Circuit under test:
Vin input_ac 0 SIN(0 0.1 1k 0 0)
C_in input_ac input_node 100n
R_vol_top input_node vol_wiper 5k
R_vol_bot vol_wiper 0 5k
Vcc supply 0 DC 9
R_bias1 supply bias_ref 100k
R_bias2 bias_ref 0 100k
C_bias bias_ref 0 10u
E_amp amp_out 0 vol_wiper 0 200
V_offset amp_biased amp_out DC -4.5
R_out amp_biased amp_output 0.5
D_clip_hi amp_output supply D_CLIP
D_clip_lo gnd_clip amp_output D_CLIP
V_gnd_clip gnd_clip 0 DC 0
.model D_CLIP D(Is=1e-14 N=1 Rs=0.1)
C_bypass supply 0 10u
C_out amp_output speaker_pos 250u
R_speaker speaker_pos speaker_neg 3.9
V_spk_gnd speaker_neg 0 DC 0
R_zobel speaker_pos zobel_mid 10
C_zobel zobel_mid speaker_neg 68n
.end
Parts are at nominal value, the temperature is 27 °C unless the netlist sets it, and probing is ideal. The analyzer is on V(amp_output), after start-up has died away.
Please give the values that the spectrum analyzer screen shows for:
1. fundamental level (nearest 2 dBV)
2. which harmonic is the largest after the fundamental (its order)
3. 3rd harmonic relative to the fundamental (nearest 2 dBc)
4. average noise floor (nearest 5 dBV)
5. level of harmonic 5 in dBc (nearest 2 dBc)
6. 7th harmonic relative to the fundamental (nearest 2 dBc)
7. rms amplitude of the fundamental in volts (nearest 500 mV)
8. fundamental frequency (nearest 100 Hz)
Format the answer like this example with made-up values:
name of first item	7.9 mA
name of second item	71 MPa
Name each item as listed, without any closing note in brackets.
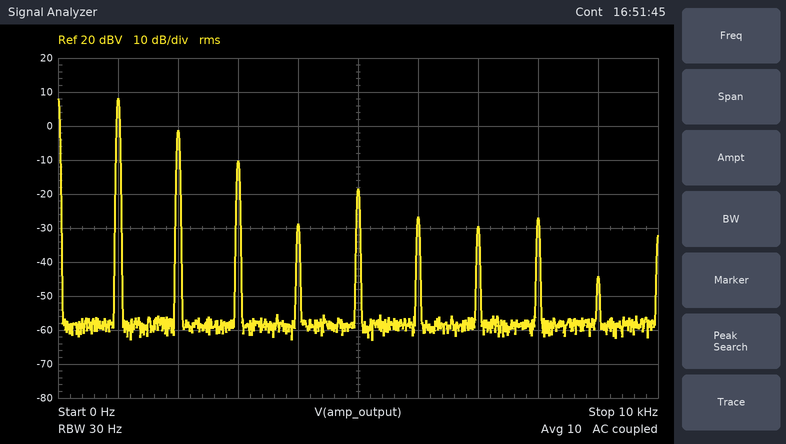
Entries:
fundamental level	8 dBV
which harmonic is the largest after the fundamental	2
3rd harmonic relative to the fundamental	-18 dBc
average noise floor	-60 dBV
level of harmonic 5 in dBc	-26 dBc
7th harmonic relative to the fundamental	-38 dBc
rms amplitude of the fundamental in volts	2.5 V
fundamental frequency	1.0 kHz
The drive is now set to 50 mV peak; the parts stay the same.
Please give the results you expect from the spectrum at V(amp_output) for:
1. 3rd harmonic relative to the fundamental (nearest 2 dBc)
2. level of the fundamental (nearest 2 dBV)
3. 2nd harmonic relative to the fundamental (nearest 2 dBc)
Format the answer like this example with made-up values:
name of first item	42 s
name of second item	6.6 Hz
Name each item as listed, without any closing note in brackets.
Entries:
3rd harmonic relative to the fundamental	-16 dBc
level of the fundamental	-2 dBV
2nd harmonic relative to the fundamental	-14 dBc
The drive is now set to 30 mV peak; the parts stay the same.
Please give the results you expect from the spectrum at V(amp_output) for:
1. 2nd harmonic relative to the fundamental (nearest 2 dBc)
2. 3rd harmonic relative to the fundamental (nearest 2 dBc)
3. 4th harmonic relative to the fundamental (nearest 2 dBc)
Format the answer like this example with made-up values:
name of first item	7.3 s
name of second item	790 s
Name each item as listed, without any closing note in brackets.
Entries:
2nd harmonic relative to the fundamental	-40 dBc
3rd harmonic relative to the fundamental	-50 dBc
4th harmonic relative to the fundamental	-58 dBc
